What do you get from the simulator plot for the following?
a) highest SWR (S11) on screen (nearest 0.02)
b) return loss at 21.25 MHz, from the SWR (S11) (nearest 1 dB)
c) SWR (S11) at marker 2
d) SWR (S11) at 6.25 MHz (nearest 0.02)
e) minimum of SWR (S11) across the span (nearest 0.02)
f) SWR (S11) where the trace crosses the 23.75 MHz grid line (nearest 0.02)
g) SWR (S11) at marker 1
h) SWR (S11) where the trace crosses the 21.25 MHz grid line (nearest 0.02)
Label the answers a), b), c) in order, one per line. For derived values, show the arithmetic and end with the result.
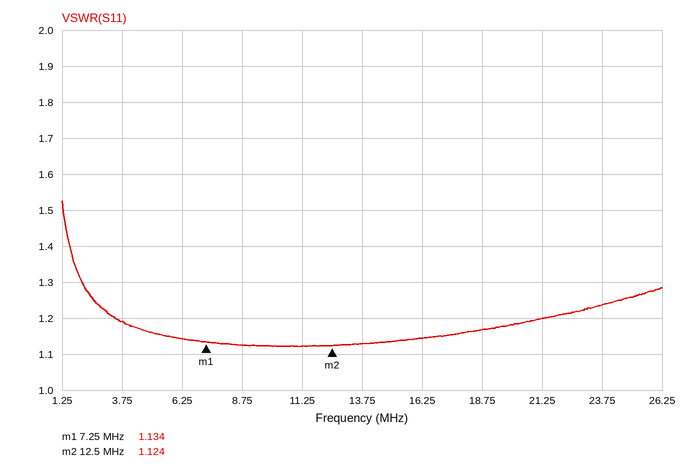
a) 1.52
b) −20 log10((1.2 − 1)/(1.2 + 1)) ≈ 21 dB
c) 1.124
d) 1.14
e) 1.12
f) 1.24
g) 1.134
h) 1.20
